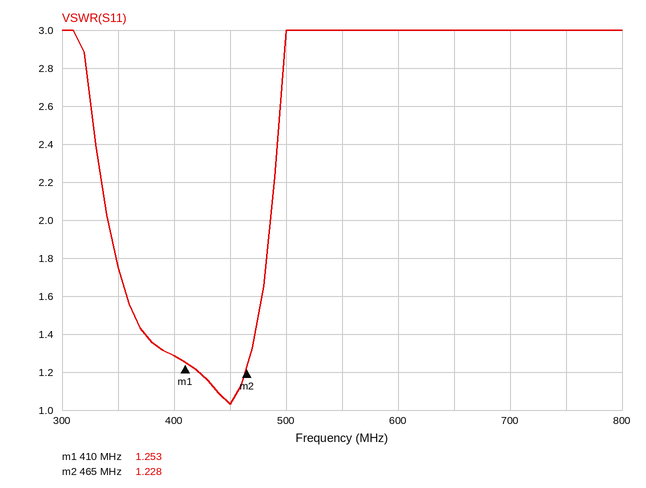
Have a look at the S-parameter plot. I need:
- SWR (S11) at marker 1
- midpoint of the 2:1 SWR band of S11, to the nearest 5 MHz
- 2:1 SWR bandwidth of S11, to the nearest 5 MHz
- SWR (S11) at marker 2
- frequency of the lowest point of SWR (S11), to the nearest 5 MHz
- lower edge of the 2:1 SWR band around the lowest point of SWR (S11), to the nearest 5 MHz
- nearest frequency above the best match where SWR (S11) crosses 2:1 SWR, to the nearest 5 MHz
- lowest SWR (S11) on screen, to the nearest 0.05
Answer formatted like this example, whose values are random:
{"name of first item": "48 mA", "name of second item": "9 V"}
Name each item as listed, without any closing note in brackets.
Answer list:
{"SWR (S11) at marker 1": "1.253", "midpoint of the 2:1 SWR band of S11, to the nearest 5 MHz": "415 MHz", "2:1 SWR bandwidth of S11, to the nearest 5 MHz": "145 MHz", "SWR (S11) at marker 2": "1.228", "frequency of the lowest point of SWR (S11), to the nearest 5 MHz": "450 MHz", "lower edge of the 2:1 SWR band around the lowest point of SWR (S11), to the nearest 5 MHz": "340 MHz", "nearest frequency above the best match where SWR (S11) crosses 2:1 SWR, to the nearest 5 MHz": "485 MHz", "lowest SWR (S11) on screen, to the nearest 0.05": "1.05"}
